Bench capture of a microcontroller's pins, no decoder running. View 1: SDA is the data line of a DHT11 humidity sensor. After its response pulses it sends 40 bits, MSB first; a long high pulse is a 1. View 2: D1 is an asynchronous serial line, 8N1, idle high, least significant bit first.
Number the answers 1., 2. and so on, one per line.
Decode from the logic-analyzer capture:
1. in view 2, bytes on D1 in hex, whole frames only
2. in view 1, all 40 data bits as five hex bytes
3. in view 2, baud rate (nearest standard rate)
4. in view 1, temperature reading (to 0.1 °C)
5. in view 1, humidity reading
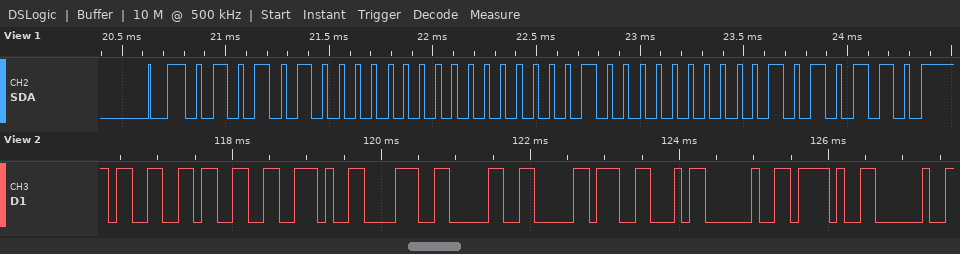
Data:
1. 0x33 0x33 0x2E 0x38 0x30 0xB0 0x46 0x20 0x2F 0x20
2. 54 00 02 00 56
3. 9600 baud
4. 2.0 °C
5. 84 %
